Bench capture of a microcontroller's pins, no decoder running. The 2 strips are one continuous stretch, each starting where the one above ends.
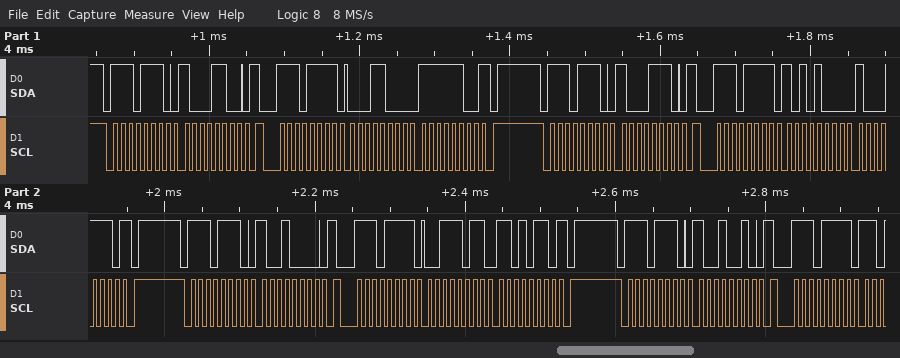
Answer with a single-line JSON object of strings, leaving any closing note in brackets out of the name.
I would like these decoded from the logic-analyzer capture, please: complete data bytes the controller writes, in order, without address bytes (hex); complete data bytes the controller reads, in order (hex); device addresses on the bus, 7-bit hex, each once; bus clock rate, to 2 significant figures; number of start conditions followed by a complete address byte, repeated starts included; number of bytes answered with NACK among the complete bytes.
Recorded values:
{"complete data bytes the controller writes, in order, without address bytes": "8C 8E 90 92", "complete data bytes the controller reads, in order": "18 FC A8 8E 3B D6", "device addresses on the bus, 7-bit hex, each once": "0x77", "bus clock rate, to 2 significant figures": "100 kHz", "number of start conditions followed by a complete address byte, repeated starts included": "8", "number of bytes answered with NACK among the complete bytes": "3"}
